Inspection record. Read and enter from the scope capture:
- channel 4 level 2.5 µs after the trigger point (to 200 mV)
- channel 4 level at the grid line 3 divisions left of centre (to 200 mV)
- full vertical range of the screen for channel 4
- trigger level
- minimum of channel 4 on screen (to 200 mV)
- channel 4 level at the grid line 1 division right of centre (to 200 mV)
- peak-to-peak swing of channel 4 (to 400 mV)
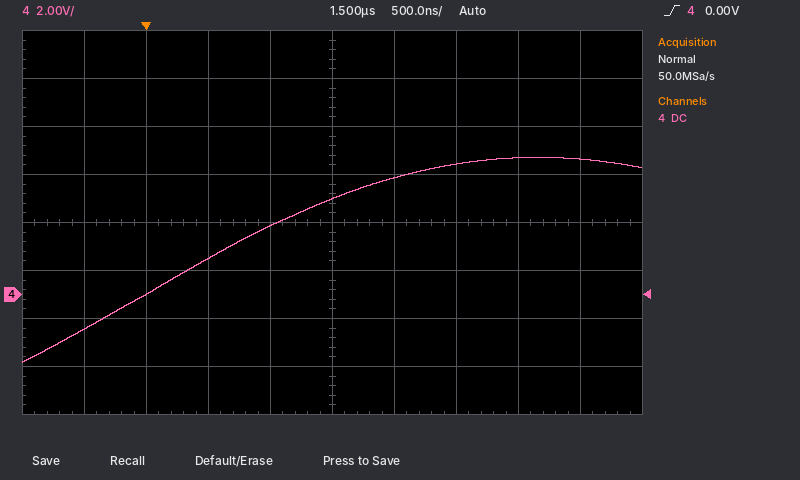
5.4 V
0.0 V
16 V
0.00 V
-2.8 V
4.8 V
8.4 V
